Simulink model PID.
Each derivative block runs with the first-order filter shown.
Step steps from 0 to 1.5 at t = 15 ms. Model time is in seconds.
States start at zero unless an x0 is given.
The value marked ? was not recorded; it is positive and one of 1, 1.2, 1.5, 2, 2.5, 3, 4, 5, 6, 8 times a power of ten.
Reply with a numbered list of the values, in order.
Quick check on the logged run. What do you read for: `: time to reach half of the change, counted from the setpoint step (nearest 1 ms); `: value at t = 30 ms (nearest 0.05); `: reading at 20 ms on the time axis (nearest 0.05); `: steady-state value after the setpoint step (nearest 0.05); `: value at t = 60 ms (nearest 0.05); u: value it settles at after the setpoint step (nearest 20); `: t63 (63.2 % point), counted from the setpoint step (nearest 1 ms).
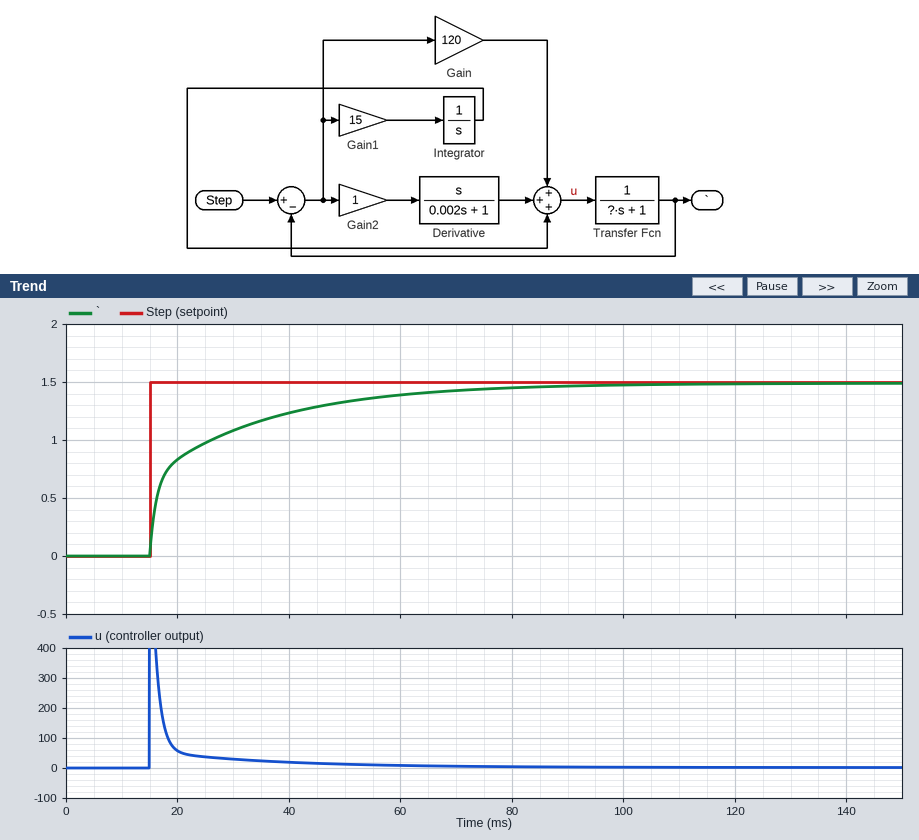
1. 3 ms
2. 1.10
3. 0.85
4. 1.50
5. 1.40
6. 0
7. 9 ms
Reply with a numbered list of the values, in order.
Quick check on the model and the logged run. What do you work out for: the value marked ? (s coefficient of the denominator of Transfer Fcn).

1. 1.5
